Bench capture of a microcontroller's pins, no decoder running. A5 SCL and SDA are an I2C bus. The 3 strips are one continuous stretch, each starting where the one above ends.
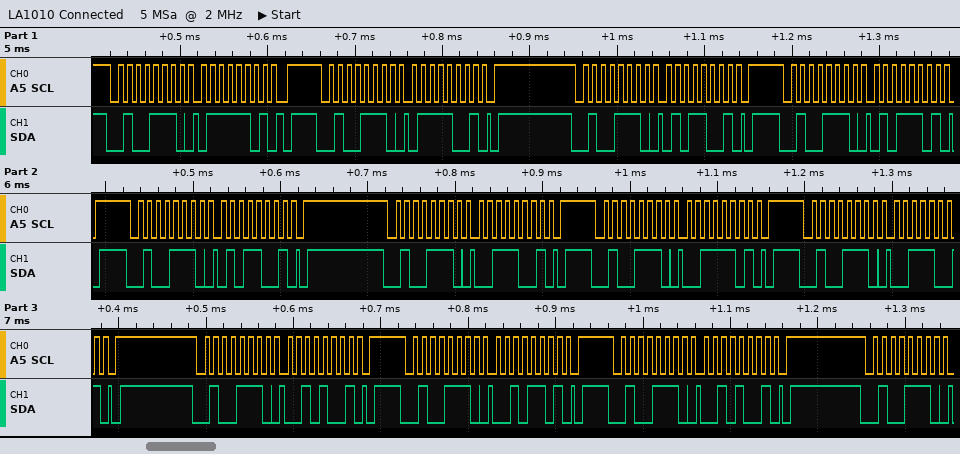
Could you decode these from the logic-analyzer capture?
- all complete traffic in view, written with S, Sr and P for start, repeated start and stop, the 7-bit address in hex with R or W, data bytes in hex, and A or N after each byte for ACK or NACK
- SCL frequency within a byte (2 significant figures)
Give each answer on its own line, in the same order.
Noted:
S 27W A 7D A P S 27W A 79 A P S 27W A 59 A P S 27W A 5D A P S 27W A 59 A P S 27W A 39 A P S 27W A 3D A P S 27W A 39 A P S 27W A 29 A P S 27W A 2D A P S 27W A 29 A P S 27W A
100 kHz
